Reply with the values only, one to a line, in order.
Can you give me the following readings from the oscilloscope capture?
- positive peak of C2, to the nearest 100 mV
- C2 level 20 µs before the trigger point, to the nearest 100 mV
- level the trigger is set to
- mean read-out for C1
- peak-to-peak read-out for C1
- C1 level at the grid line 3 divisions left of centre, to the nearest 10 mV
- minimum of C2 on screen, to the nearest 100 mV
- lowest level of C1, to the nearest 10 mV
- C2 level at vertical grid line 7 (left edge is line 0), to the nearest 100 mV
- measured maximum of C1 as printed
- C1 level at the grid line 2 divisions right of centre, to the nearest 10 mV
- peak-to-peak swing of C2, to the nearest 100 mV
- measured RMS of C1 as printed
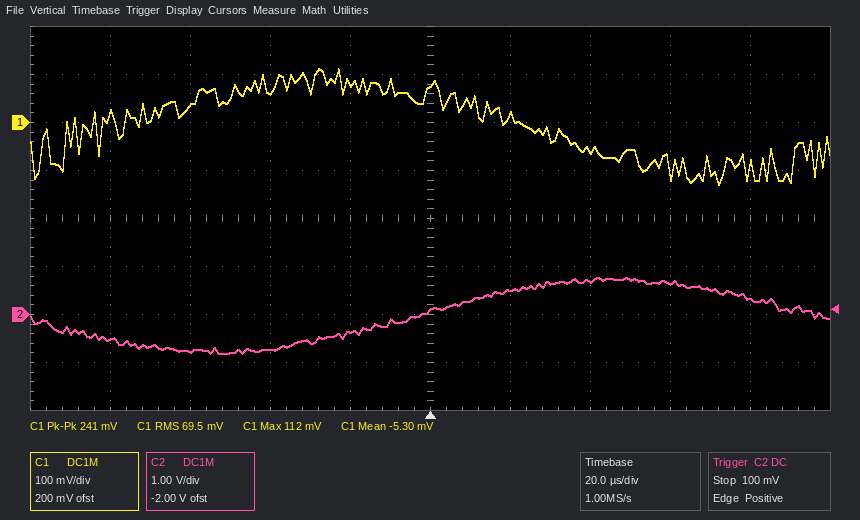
800 mV
-400 mV
100 mV
-5.30 mV
241 mV
30 mV
-800 mV
-130 mV
700 mV
112 mV
-60 mV
1.6 V
69.5 mV
